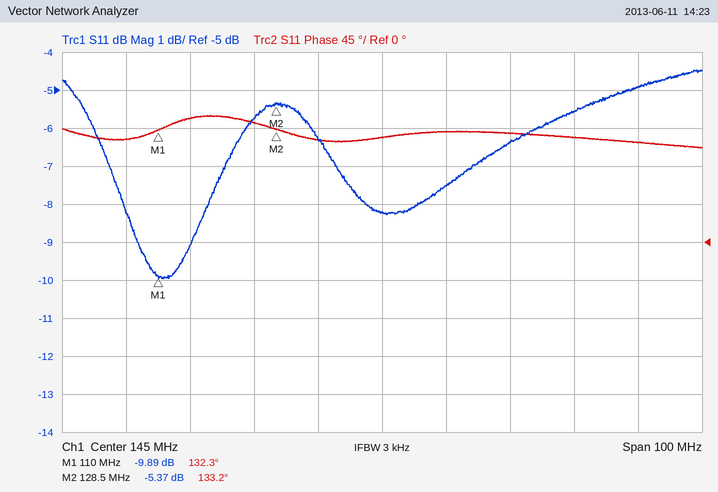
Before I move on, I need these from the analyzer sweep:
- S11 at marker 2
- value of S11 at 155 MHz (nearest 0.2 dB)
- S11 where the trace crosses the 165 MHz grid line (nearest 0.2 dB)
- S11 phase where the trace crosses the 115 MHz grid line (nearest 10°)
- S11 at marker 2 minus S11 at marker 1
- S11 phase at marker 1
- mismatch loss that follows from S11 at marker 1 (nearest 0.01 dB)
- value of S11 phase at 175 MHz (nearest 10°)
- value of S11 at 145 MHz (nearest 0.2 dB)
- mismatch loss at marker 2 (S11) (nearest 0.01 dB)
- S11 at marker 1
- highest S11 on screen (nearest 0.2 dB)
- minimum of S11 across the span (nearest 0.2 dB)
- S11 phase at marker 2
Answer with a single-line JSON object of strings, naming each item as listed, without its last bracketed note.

{"S11 at marker 2": "-5.37 dB", "value of S11 at 155 MHz": "-7.6 dB", "S11 where the trace crosses the 165 MHz grid line": "-6.4 dB", "S11 phase where the trace crosses the 115 MHz grid line": "150°", "S11 at marker 2 minus S11 at marker 1": "4.52 dB", "S11 phase at marker 1": "132.3°", "mismatch loss that follows from S11 at marker 1": "0.47 dB", "value of S11 phase at 175 MHz": "120°", "value of S11 at 145 MHz": "-8.2 dB", "mismatch loss at marker 2 (S11)": "1.49 dB", "S11 at marker 1": "-9.89 dB", "highest S11 on screen": "-4.4 dB", "minimum of S11 across the span": "-10.0 dB", "S11 phase at marker 2": "133.2°"}
